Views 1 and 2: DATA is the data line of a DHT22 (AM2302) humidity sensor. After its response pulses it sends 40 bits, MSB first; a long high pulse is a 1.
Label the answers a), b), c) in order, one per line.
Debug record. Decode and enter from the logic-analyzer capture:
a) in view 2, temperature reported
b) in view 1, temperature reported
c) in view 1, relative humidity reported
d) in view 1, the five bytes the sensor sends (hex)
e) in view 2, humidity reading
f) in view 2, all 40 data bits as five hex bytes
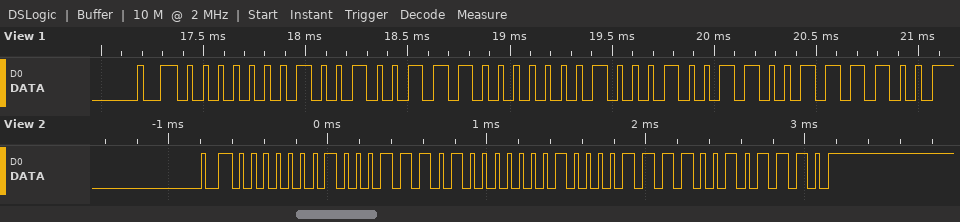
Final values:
a) 27.1 °C
b) 27.5 °C
c) 29.5 %
d) 01 27 01 13 3C
e) 28.5 %
f) 01 1D 01 0F 2E
